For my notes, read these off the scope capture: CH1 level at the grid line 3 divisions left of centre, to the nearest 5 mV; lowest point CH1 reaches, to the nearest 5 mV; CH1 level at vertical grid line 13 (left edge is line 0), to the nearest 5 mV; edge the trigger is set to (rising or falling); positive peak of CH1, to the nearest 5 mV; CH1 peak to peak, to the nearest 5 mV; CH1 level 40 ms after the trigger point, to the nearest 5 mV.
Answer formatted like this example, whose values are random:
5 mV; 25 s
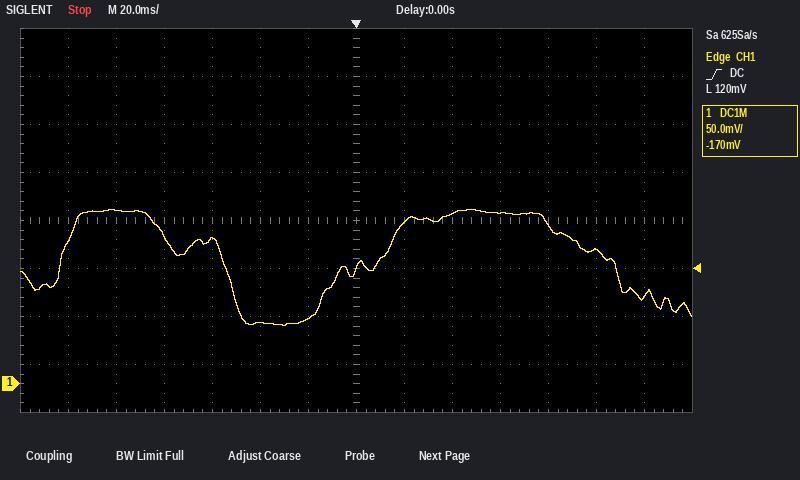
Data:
150 mV; 60 mV; 90 mV; rising; 180 mV; 120 mV; 175 mV
